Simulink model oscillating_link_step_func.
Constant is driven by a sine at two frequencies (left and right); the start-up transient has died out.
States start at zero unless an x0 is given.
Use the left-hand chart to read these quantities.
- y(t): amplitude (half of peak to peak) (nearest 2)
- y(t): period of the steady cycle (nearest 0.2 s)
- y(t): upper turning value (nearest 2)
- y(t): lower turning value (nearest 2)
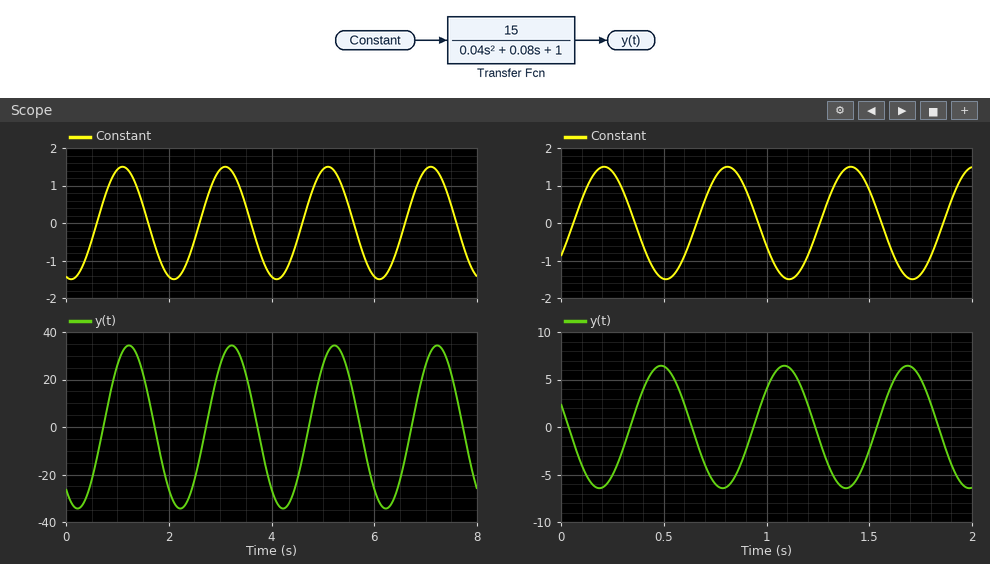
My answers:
34
2.0 s
34
-34
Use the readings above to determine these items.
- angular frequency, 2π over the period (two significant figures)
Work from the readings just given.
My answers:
3.1 rad/s
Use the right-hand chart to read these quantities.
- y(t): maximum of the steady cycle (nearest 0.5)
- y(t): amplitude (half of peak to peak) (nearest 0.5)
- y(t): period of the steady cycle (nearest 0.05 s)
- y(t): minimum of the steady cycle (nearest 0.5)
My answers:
6.5
6.5
0.60 s
-6.5
